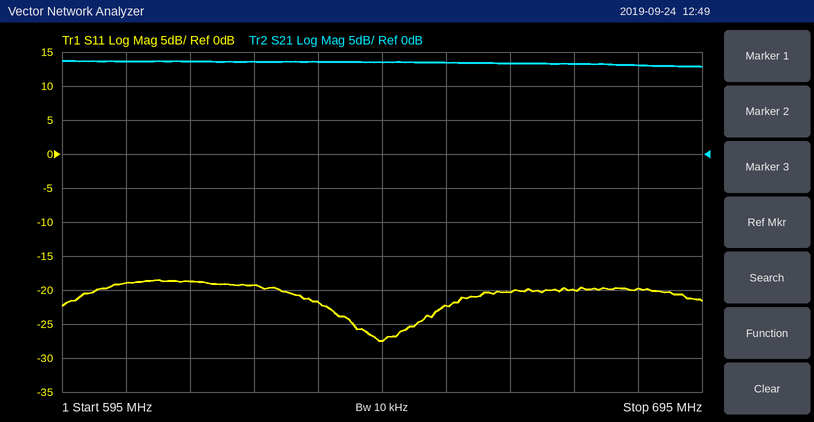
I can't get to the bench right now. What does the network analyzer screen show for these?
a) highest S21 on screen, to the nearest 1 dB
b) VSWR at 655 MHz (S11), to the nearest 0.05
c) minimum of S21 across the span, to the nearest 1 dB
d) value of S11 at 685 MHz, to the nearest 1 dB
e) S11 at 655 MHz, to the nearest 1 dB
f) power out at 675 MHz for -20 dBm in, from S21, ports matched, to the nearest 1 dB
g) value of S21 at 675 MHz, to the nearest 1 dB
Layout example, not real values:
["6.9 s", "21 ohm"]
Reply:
["14 dB", "1.15", "13 dB", "-20 dB", "-22 dB", "-7 dBm", "13 dB"]
